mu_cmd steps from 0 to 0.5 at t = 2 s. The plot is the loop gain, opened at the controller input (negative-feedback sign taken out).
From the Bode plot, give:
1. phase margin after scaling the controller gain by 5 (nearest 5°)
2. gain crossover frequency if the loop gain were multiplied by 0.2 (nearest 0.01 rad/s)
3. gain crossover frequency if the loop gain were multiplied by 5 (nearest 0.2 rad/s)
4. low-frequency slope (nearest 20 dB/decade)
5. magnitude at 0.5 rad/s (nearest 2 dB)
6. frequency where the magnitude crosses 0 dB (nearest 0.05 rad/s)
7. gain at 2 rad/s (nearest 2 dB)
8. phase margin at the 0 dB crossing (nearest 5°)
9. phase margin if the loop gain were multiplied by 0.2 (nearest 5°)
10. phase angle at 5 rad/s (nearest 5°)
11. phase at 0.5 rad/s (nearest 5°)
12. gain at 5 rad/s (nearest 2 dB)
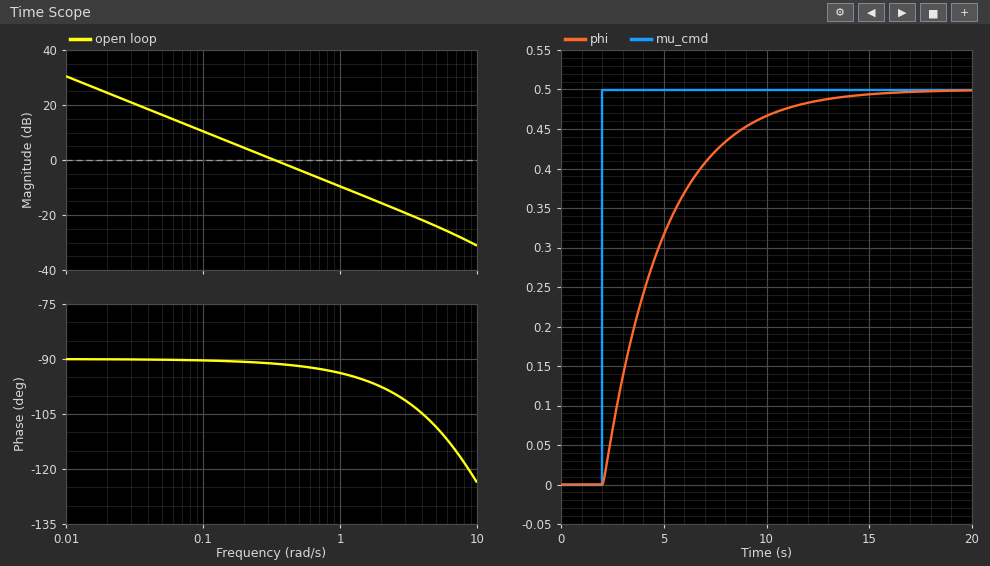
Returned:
85°
0.07 rad/s
1.6 rad/s
-20 dB/decade
-4 dB
0.35 rad/s
-16 dB
90°
90°
-110°
-90°
-24 dB
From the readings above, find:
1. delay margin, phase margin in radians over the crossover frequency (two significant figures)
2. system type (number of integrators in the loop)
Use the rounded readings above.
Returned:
4.5 s
1
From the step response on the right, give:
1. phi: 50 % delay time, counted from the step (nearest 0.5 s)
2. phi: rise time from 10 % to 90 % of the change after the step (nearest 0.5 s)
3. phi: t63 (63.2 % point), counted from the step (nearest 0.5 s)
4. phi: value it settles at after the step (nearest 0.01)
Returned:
2.0 s
6.5 s
3.0 s
0.50
